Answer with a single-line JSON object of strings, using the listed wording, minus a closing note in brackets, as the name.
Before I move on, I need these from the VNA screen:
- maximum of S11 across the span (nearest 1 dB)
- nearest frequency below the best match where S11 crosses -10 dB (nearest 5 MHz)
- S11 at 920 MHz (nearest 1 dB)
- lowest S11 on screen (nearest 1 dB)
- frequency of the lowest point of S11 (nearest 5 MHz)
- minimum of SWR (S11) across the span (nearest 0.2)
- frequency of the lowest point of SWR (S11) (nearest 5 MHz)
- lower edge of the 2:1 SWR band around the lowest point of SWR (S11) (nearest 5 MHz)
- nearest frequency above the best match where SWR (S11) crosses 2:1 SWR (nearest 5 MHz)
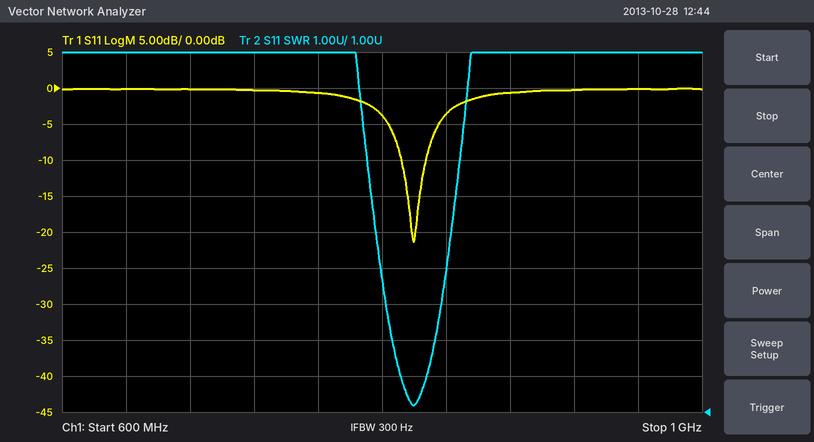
{"maximum of S11 across the span": "0 dB", "nearest frequency below the best match where S11 crosses -10 dB": "810 MHz", "S11 at 920 MHz": "0 dB", "lowest S11 on screen": "-21 dB", "frequency of the lowest point of S11": "820 MHz", "minimum of SWR (S11) across the span": "1.2", "frequency of the lowest point of SWR (S11)": "820 MHz", "lower edge of the 2:1 SWR band around the lowest point of SWR (S11)": "810 MHz", "nearest frequency above the best match where SWR (S11) crosses 2:1 SWR": "830 MHz"}
